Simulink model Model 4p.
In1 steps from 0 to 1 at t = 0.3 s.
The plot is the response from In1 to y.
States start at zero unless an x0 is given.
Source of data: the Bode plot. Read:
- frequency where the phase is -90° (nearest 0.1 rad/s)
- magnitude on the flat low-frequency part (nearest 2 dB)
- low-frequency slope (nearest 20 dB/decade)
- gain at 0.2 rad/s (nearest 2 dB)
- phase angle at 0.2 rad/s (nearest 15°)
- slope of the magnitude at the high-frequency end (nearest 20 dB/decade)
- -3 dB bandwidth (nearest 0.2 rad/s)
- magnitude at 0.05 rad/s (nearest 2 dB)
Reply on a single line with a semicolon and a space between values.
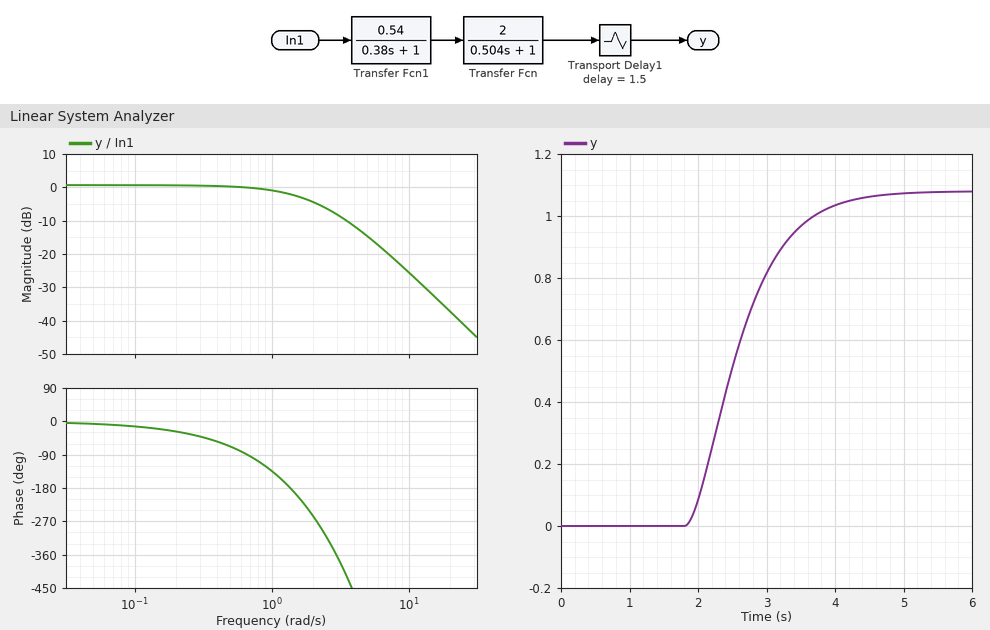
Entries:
0.7 rad/s; 0 dB; 0 dB/decade; 0 dB; -30°; -40 dB/decade; 1.4 rad/s; 0 dB
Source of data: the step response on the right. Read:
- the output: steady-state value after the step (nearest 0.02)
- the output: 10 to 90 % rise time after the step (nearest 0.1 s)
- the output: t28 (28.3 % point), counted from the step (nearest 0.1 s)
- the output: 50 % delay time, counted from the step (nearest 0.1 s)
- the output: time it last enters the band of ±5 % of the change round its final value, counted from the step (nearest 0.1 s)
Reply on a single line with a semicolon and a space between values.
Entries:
1.08; 1.5 s; 2.0 s; 2.2 s; 3.6 s
